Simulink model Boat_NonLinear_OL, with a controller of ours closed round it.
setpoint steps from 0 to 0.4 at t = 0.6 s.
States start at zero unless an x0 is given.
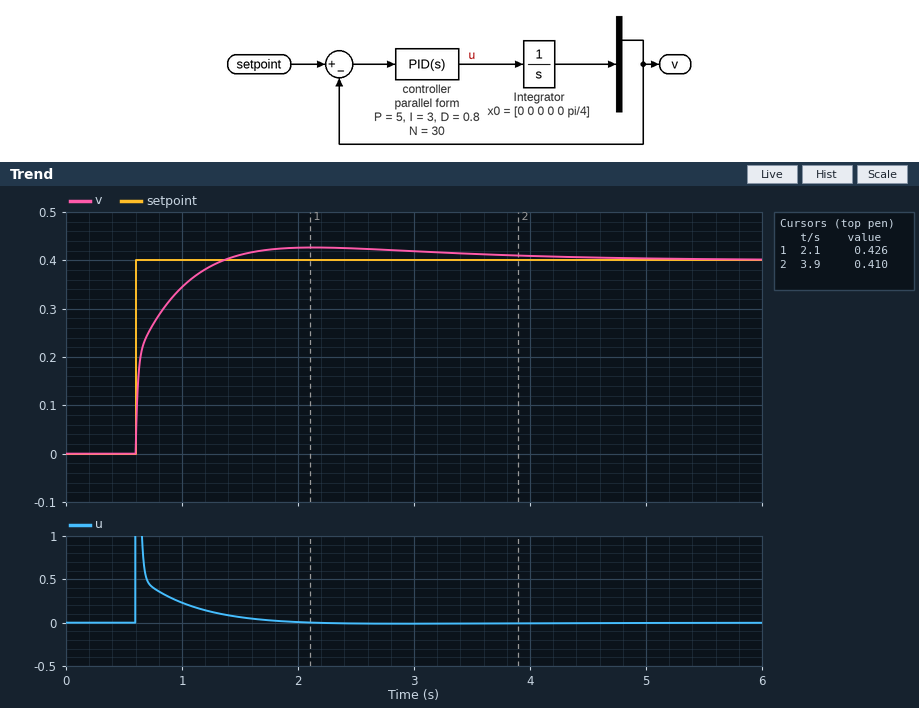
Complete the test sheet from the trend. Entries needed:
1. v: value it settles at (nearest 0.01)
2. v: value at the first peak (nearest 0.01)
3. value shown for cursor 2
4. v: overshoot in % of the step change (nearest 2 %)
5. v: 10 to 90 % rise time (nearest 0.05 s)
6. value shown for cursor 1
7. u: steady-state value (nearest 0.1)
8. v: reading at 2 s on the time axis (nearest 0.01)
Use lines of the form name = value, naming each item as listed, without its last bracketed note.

v: value it settles at = 0.40
v: value at the first peak = 0.43
value shown for cursor 2 = 0.410
v: overshoot in % of the step change = 6 %
v: 10 to 90 % rise time = 0.45 s
value shown for cursor 1 = 0.426
u: steady-state value = 0.0
v: reading at 2 s on the time axis = 0.43
